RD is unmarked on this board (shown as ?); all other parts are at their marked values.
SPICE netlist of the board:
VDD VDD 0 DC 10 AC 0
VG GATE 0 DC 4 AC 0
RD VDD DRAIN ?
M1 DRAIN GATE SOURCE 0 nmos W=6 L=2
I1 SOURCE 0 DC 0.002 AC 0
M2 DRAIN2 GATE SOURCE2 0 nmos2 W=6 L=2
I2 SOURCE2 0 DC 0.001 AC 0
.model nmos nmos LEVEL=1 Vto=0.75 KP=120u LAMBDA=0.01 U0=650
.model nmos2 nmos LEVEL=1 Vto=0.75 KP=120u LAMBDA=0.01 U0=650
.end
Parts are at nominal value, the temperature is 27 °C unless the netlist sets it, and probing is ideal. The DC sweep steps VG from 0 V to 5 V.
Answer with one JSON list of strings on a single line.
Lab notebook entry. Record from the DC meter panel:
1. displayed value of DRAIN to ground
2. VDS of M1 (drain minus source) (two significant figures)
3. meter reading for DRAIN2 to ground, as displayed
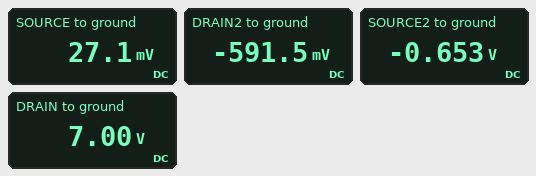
["7.00 V", "7.0 V", "-591.5 mV"]
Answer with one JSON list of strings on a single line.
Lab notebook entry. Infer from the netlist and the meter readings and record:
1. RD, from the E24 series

["1.5 kΩ"]
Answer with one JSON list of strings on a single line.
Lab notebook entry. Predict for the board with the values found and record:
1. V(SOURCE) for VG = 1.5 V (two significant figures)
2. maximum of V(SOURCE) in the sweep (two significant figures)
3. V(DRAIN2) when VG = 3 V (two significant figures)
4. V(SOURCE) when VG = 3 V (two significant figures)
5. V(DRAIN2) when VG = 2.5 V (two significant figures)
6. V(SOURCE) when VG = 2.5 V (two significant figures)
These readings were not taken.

["-670 mV", "1.0 V", "-590 mV", "-630 mV", "-580 mV", "-650 mV"]
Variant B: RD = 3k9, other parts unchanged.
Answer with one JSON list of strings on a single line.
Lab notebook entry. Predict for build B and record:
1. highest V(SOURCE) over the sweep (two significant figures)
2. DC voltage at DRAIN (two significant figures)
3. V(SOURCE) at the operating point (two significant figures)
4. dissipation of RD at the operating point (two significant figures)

["360 mV", "2.2 V", "-210 mV", "16 mW"]
